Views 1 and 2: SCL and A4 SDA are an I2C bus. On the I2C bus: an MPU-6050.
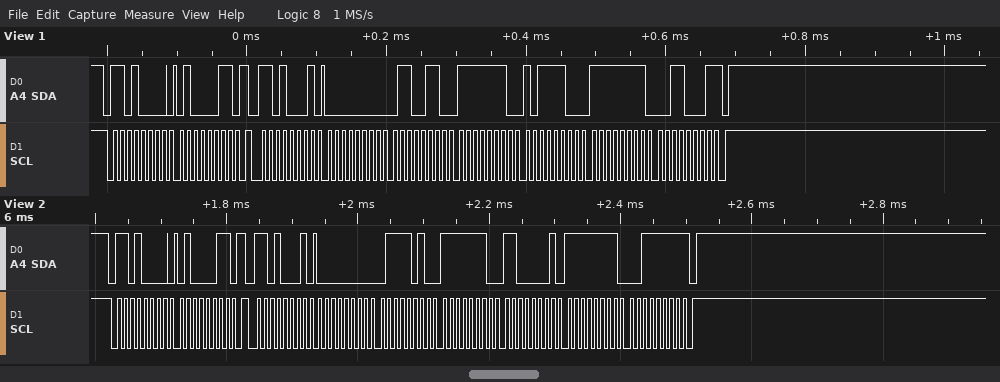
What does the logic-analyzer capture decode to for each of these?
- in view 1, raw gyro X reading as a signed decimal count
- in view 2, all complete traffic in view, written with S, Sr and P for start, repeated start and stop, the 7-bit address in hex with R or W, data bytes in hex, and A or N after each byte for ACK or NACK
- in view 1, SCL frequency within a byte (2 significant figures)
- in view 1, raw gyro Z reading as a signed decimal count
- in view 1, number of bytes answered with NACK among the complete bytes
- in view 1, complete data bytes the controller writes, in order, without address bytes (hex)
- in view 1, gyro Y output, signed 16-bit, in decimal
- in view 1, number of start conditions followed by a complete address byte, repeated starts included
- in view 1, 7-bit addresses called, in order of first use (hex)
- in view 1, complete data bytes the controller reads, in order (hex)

102
S 68W A 43 A Sr 68R A 00 A 7A A FE A C1 A FF A 3F N P
100 kHz
-207
1
43
-324
2
0x68
00 66 FE BC FF 31
